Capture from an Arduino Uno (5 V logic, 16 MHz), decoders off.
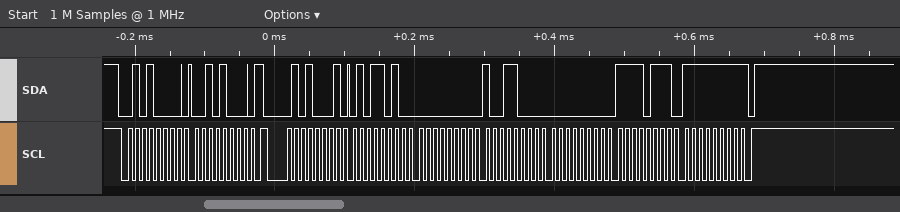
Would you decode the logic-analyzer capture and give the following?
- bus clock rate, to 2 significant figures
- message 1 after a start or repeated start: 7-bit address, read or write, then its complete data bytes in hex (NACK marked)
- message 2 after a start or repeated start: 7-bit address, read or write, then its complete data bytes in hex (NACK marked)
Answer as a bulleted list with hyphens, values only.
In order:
- 100 kHz
- 0x28 write: 28
- 0x28 read: 5A 00 98 00 F7 FF NACK
